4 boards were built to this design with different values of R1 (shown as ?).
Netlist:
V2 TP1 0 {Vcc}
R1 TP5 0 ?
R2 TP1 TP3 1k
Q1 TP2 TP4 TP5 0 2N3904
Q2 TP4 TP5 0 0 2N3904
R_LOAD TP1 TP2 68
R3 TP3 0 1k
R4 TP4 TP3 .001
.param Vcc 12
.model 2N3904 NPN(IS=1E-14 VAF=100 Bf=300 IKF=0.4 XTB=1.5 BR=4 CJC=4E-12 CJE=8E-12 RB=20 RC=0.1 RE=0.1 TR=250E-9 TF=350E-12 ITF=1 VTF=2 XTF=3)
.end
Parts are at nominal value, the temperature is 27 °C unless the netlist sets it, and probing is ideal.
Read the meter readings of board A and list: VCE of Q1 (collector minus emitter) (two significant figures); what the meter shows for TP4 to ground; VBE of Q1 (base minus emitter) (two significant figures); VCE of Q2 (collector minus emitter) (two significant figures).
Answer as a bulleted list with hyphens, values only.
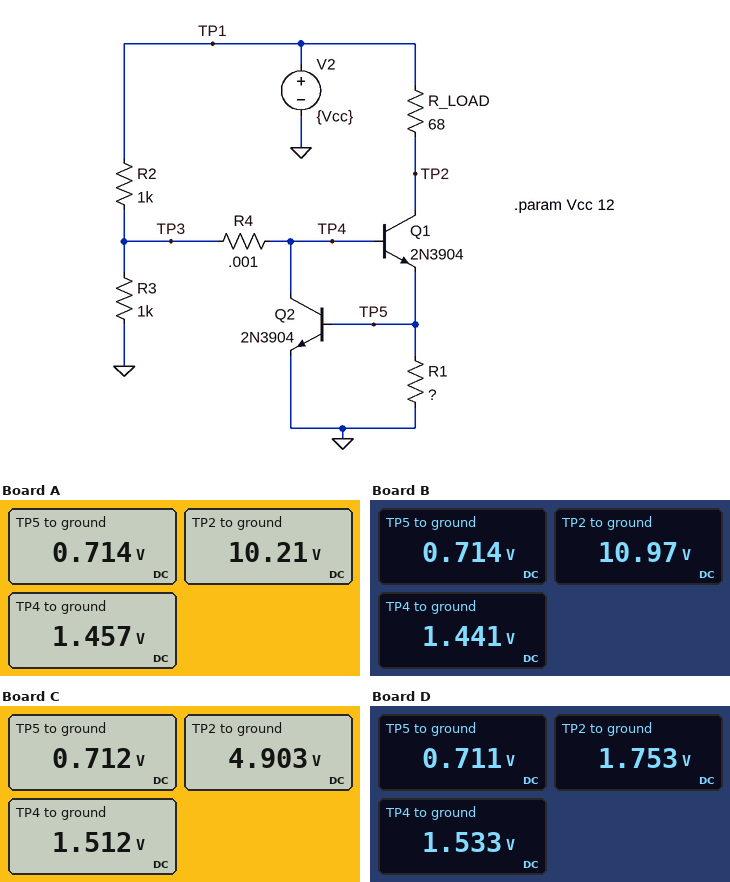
- 9.5 V
- 1.457 V
- 740 mV
- 1.5 V
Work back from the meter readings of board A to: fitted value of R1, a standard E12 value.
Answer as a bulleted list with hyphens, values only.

- 27 Ω
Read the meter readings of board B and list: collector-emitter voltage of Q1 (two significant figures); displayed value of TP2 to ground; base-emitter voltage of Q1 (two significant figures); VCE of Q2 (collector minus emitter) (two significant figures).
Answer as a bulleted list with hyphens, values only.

- 10 V
- 10.97 V
- 730 mV
- 1.4 V
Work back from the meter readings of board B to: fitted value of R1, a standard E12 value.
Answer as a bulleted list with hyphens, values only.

- 47 Ω
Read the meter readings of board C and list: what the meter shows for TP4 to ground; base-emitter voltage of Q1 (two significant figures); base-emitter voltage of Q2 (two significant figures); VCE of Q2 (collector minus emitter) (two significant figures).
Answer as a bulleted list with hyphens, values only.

- 1.512 V
- 800 mV
- 710 mV
- 1.5 V
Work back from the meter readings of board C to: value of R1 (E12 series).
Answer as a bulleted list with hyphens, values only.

- 6.8 Ω
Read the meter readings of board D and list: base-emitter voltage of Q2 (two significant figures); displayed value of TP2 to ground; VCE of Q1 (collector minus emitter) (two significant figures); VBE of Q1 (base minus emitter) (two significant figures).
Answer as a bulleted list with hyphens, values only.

- 710 mV
- 1.753 V
- 1.0 V
- 820 mV
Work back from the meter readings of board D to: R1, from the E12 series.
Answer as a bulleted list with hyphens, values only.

- 4.7 Ω
